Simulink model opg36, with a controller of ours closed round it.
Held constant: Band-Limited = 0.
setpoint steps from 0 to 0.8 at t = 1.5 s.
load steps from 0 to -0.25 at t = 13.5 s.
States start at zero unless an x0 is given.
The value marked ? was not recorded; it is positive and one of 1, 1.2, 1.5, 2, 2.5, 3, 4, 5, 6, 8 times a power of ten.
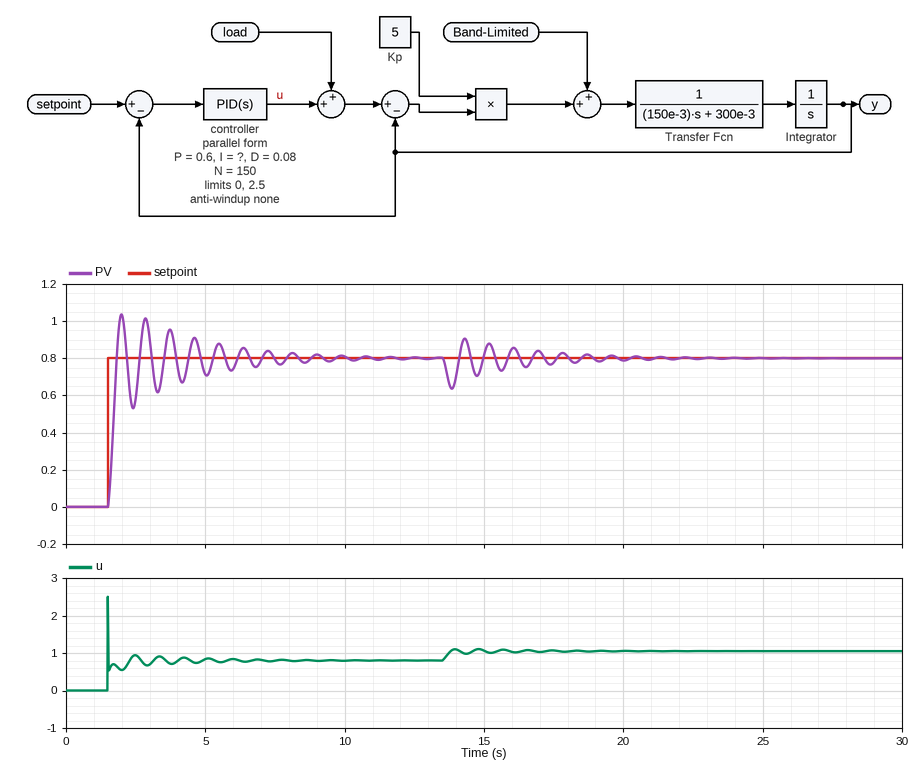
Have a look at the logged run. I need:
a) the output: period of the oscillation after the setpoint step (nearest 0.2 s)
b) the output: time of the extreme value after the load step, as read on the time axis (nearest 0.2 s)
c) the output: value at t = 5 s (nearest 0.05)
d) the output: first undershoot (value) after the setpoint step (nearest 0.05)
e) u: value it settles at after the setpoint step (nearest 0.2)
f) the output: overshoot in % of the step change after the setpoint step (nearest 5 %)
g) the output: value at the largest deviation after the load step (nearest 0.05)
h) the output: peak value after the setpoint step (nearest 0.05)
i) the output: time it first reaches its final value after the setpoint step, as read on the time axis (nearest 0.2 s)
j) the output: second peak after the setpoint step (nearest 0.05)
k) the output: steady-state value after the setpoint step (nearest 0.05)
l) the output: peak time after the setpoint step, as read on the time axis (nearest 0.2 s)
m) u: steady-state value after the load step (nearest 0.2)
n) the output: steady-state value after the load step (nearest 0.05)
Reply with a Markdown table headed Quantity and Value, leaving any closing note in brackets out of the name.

| Quantity | Value |
|---|---|
| the output: period of the oscillation after the setpoint step | 0.8 s |
| the output: time of the extreme value after the load step, as read on the time axis | 13.8 s |
| the output: value at t = 5 s | 0.70 |
| the output: first undershoot (value) after the setpoint step | 0.55 |
| u: value it settles at after the setpoint step | 0.8 |
| the output: overshoot in % of the step change after the setpoint step | 30 % |
| the output: value at the largest deviation after the load step | 0.65 |
| the output: peak value after the setpoint step | 1.05 |
| the output: time it first reaches its final value after the setpoint step, as read on the time axis | 1.8 s |
| the output: second peak after the setpoint step | 1.00 |
| the output: steady-state value after the setpoint step | 0.80 |
| the output: peak time after the setpoint step, as read on the time axis | 2.0 s |
| u: steady-state value after the load step | 1.0 |
| the output: steady-state value after the load step | 0.80 |
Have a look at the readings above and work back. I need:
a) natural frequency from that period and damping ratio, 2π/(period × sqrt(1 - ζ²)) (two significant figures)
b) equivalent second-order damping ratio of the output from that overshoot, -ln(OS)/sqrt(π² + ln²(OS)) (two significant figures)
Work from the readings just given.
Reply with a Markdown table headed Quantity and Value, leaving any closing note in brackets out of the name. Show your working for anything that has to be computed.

| Quantity | Value |
|---|---|
| natural frequency from that period and damping ratio, 2π/(period × sqrt(1 - ζ²)) | 2π / (0.8 × sqrt(1 - 0.36²)) = 8.4 rad/s |
| equivalent second-order damping ratio of the output from that overshoot, -ln(OS)/sqrt(π² + ln²(OS)) | ln(0.3) = -1.204; 1.204 / sqrt(9.870 + 1.450) = 0.36 |
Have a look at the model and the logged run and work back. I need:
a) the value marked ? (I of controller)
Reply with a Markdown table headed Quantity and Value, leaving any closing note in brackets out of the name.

| Quantity | Value |
|---|---|
| the value marked ? | 6 |
